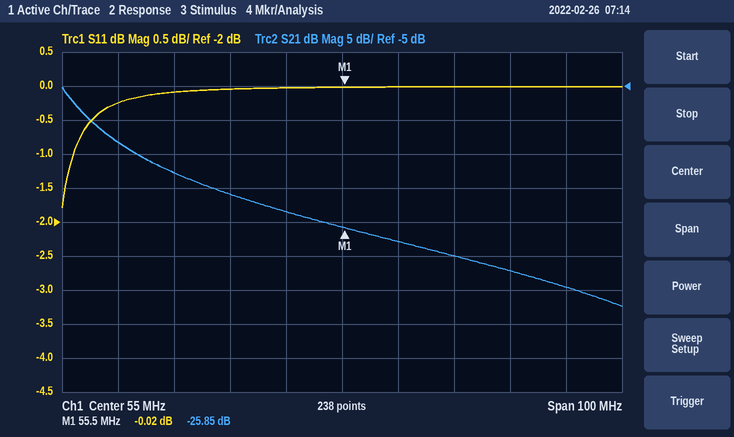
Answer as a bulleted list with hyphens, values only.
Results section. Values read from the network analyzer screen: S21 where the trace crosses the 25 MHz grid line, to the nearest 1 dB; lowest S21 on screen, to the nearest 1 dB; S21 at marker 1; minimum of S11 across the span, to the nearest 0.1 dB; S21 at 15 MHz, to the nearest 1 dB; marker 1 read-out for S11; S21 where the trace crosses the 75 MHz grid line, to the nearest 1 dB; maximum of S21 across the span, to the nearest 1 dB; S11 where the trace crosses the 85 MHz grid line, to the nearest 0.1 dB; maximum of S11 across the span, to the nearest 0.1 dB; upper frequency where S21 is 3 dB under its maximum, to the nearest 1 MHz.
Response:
- -18 dB
- -37 dB
- -25.85 dB
- -1.8 dB
- -13 dB
- -0.02 dB
- -30 dB
- -5 dB
- 0.0 dB
- 0.0 dB
- 8 MHz
